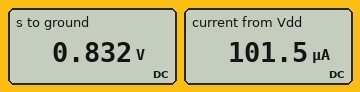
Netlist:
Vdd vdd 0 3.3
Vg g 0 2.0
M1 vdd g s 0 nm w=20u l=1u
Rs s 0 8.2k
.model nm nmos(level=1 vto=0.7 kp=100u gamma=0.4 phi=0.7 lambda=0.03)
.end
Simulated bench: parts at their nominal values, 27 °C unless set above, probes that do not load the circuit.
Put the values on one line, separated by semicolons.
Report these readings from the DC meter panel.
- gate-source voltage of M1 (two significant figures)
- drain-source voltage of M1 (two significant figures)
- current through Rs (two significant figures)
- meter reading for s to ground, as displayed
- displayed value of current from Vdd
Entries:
1.2 V; 2.5 V; 100 µA; 0.832 V; 101.5 µA
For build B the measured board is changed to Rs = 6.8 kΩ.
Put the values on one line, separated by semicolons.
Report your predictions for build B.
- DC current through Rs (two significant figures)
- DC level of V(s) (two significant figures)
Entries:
120 µA; 810 mV
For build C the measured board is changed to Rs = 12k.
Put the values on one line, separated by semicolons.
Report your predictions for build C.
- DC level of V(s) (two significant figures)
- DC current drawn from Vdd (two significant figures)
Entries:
870 mV; 73 µA
